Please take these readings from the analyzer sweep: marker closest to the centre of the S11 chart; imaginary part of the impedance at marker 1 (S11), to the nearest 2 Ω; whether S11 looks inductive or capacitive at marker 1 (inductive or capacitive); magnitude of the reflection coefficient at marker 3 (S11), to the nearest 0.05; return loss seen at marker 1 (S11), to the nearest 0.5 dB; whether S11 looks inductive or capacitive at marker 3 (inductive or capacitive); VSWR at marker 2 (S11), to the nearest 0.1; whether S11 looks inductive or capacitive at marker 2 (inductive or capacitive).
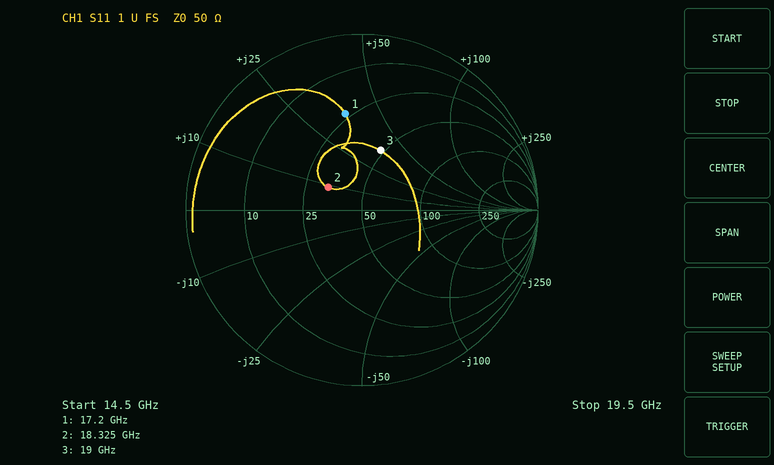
marker 2
+36 Ω
inductive
0.35
5.0 dB
inductive
1.6
inductive
